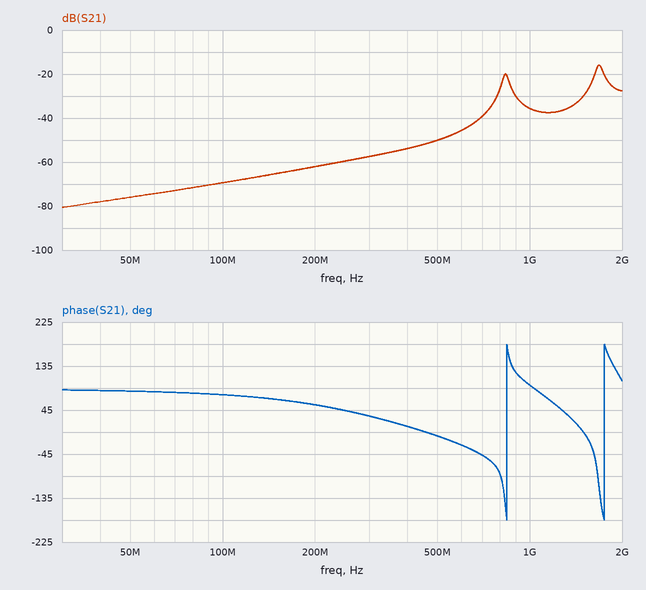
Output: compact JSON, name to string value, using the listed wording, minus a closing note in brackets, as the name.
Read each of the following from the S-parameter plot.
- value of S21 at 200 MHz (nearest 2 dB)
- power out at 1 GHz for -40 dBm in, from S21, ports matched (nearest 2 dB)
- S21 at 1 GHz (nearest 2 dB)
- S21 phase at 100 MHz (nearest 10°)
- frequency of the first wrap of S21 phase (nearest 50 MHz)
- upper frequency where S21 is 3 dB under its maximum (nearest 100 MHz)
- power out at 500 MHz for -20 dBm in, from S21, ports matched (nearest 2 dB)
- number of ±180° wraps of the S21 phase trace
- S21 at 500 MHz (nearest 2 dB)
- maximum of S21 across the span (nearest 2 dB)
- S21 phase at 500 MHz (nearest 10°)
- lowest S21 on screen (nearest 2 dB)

{"value of S21 at 200 MHz": "-62 dB", "power out at 1 GHz for -40 dBm in, from S21, ports matched": "-76 dBm", "S21 at 1 GHz": "-36 dB", "S21 phase at 100 MHz": "80°", "frequency of the first wrap of S21 phase": "850 MHz", "upper frequency where S21 is 3 dB under its maximum": "1.7 GHz", "power out at 500 MHz for -20 dBm in, from S21, ports matched": "-70 dBm", "number of ±180° wraps of the S21 phase trace": "2", "S21 at 500 MHz": "-50 dB", "maximum of S21 across the span": "-16 dB", "S21 phase at 500 MHz": "-10°", "lowest S21 on screen": "-80 dB"}
